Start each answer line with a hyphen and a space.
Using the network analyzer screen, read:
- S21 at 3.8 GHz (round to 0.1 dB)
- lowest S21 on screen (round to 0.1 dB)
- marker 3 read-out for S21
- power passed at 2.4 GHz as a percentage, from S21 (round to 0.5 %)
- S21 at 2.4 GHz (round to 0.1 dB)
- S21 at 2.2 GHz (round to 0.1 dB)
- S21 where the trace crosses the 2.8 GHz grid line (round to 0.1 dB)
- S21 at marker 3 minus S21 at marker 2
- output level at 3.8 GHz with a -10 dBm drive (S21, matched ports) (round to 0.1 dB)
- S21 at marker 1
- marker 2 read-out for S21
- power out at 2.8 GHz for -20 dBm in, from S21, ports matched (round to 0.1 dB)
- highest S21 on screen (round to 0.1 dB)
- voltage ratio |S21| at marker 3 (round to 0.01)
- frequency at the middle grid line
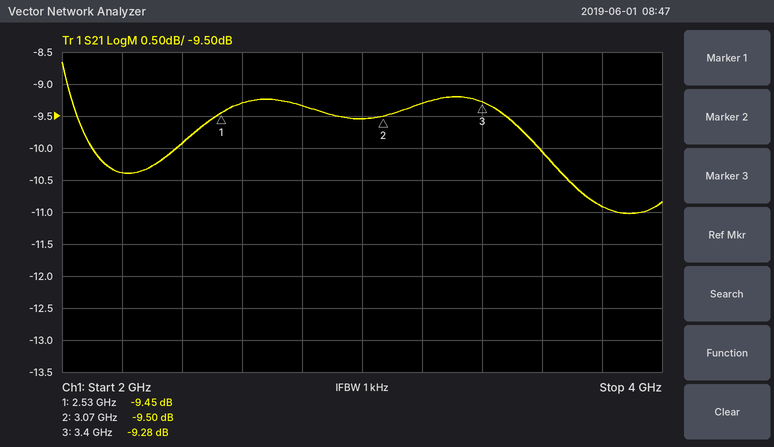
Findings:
- -10.9 dB
- -11.0 dB
- -9.28 dB
- 10.0 %
- -9.9 dB
- -10.4 dB
- -9.3 dB
- 0.22 dB
- -20.9 dBm
- -9.45 dB
- -9.50 dB
- -29.3 dBm
- -8.7 dB
- 0.34
- 3 GHz
